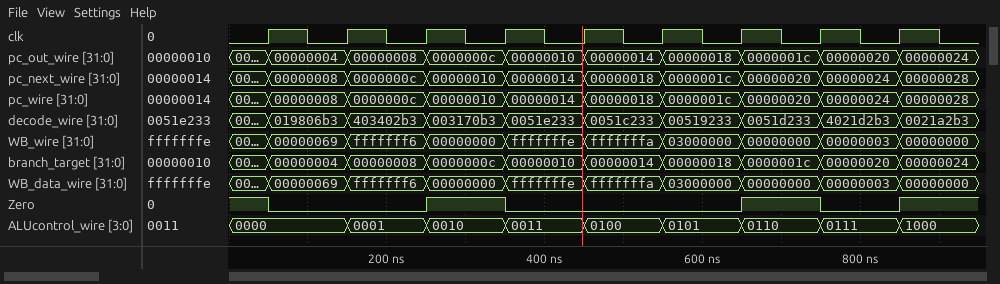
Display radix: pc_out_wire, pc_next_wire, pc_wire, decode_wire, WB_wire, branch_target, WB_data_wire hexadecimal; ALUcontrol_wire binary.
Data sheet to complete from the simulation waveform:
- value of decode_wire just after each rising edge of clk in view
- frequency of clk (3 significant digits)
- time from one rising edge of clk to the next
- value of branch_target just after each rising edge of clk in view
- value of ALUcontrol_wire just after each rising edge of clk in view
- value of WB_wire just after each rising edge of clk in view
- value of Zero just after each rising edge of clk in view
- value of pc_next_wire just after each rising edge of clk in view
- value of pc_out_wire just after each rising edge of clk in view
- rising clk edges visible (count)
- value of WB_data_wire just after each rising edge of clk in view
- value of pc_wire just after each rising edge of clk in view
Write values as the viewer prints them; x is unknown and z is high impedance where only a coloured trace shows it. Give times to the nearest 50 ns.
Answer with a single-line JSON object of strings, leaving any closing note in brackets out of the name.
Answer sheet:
{"value of decode_wire just after each rising edge of clk in view": "019806b3, 403402b3, 003170b3, 0051e233, 0051c233, 00519233, 0051d233, 4021d2b3, 0021a2b3", "frequency of clk": "10.0 MHz", "time from one rising edge of clk to the next": "100 ns", "value of branch_target just after each rising edge of clk in view": "00000004, 00000008, 0000000c, 00000010, 00000014, 00000018, 0000001c, 00000020, 00000024", "value of ALUcontrol_wire just after each rising edge of clk in view": "0000, 0001, 0010, 0011, 0100, 0101, 0110, 0111, 1000", "value of WB_wire just after each rising edge of clk in view": "00000069, fffffff6, 00000000, fffffffe, fffffffa, 03000000, 00000000, 00000003, 00000000", "value of Zero just after each rising edge of clk in view": "0 0 1 0 0 0 1 0 1", "value of pc_next_wire just after each rising edge of clk in view": "00000008, 0000000c, 00000010, 00000014, 00000018, 0000001c, 00000020, 00000024, 00000028", "value of pc_out_wire just after each rising edge of clk in view": "00000004, 00000008, 0000000c, 00000010, 00000014, 00000018, 0000001c, 00000020, 00000024", "rising clk edges visible": "9", "value of WB_data_wire just after each rising edge of clk in view": "00000069, fffffff6, 00000000, fffffffe, fffffffa, 03000000, 00000000, 00000003, 00000000", "value of pc_wire just after each rising edge of clk in view": "00000008, 0000000c, 00000010, 00000014, 00000018, 0000001c, 00000020, 00000024, 00000028"}
